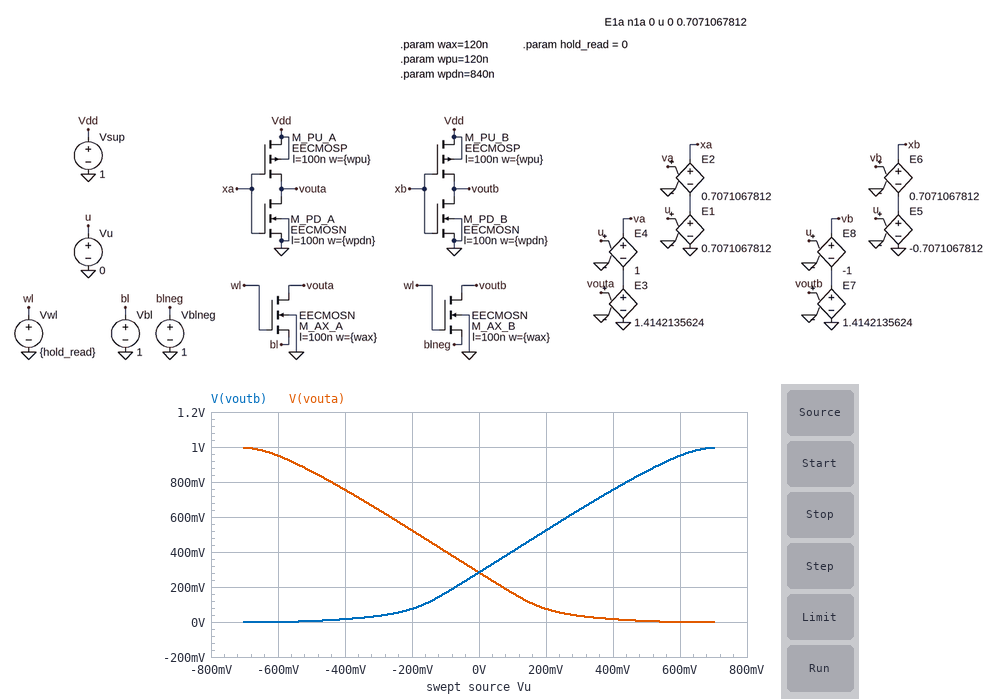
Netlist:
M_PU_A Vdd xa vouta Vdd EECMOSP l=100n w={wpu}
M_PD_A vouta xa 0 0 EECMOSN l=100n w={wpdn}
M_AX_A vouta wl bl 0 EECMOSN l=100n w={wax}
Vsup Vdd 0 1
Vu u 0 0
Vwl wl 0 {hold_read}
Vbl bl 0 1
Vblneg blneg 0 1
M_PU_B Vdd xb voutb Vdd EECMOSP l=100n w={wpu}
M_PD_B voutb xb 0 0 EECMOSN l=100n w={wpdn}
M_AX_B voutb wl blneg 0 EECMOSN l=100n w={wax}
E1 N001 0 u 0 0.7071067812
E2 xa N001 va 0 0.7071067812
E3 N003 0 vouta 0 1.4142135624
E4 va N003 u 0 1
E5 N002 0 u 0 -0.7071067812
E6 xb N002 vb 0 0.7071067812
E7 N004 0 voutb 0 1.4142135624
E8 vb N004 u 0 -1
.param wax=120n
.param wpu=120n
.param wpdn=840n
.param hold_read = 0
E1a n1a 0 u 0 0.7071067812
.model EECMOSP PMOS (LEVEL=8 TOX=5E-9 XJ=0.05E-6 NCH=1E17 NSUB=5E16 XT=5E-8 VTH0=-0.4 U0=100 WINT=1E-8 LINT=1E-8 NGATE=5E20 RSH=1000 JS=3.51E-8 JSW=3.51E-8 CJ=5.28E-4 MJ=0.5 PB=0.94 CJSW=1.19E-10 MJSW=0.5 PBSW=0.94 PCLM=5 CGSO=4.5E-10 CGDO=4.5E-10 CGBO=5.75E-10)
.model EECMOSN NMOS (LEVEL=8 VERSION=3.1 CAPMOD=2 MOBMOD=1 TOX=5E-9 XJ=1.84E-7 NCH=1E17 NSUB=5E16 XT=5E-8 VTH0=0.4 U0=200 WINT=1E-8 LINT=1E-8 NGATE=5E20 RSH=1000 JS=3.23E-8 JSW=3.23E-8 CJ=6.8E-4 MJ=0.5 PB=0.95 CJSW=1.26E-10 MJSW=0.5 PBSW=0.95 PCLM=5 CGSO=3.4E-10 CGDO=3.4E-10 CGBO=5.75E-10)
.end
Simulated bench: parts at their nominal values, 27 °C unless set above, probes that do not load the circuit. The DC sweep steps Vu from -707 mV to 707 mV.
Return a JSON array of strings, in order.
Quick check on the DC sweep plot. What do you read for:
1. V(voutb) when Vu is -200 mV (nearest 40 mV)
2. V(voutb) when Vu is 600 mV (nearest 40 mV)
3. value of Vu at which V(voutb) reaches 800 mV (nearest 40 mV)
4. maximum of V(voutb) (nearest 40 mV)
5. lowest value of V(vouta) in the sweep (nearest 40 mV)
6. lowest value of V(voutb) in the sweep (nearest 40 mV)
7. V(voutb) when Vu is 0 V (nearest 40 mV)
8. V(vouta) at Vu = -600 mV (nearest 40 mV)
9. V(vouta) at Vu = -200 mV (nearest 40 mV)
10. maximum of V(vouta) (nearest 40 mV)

["80 mV", "960 mV", "440 mV", "1.00 V", "0 V", "0 V", "280 mV", "960 mV", "520 mV", "1.00 V"]
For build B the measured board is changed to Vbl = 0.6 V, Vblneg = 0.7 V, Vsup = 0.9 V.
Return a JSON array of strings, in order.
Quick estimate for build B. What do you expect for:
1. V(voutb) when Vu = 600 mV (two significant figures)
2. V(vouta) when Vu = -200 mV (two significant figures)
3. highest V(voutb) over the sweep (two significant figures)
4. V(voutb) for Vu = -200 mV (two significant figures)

["890 mV", "510 mV", "900 mV", "58 mV"]
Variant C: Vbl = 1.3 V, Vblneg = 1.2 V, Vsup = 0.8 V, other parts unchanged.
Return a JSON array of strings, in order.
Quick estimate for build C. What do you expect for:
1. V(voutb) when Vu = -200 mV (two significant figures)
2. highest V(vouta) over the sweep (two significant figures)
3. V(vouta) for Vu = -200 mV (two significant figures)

["42 mV", "800 mV", "490 mV"]
